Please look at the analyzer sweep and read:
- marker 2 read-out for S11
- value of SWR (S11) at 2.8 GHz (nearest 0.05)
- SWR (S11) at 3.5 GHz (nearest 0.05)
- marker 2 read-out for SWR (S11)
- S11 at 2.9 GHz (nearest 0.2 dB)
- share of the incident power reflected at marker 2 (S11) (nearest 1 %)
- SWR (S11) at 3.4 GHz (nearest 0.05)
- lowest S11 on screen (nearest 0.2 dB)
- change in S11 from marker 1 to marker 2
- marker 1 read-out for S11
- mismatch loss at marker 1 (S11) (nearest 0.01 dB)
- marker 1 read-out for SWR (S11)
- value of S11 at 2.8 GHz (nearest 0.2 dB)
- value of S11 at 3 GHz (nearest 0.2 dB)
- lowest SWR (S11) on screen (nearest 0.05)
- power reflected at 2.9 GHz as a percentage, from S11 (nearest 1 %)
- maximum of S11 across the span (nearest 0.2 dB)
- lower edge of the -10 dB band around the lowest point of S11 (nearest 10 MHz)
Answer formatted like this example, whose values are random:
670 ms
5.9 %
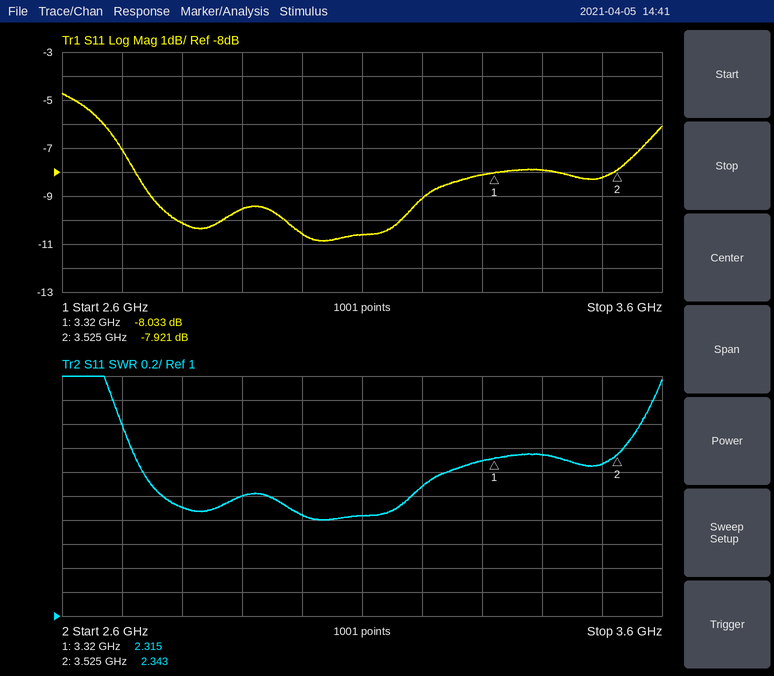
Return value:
-7.921 dB
1.90
2.25
2.343
-9.6 dB
16 %
2.35
-10.8 dB
0.112 dB
-8.033 dB
0.74 dB
2.315
-10.2 dB
-10.6 dB
1.80
11 %
-4.8 dB
2.97 GHz
